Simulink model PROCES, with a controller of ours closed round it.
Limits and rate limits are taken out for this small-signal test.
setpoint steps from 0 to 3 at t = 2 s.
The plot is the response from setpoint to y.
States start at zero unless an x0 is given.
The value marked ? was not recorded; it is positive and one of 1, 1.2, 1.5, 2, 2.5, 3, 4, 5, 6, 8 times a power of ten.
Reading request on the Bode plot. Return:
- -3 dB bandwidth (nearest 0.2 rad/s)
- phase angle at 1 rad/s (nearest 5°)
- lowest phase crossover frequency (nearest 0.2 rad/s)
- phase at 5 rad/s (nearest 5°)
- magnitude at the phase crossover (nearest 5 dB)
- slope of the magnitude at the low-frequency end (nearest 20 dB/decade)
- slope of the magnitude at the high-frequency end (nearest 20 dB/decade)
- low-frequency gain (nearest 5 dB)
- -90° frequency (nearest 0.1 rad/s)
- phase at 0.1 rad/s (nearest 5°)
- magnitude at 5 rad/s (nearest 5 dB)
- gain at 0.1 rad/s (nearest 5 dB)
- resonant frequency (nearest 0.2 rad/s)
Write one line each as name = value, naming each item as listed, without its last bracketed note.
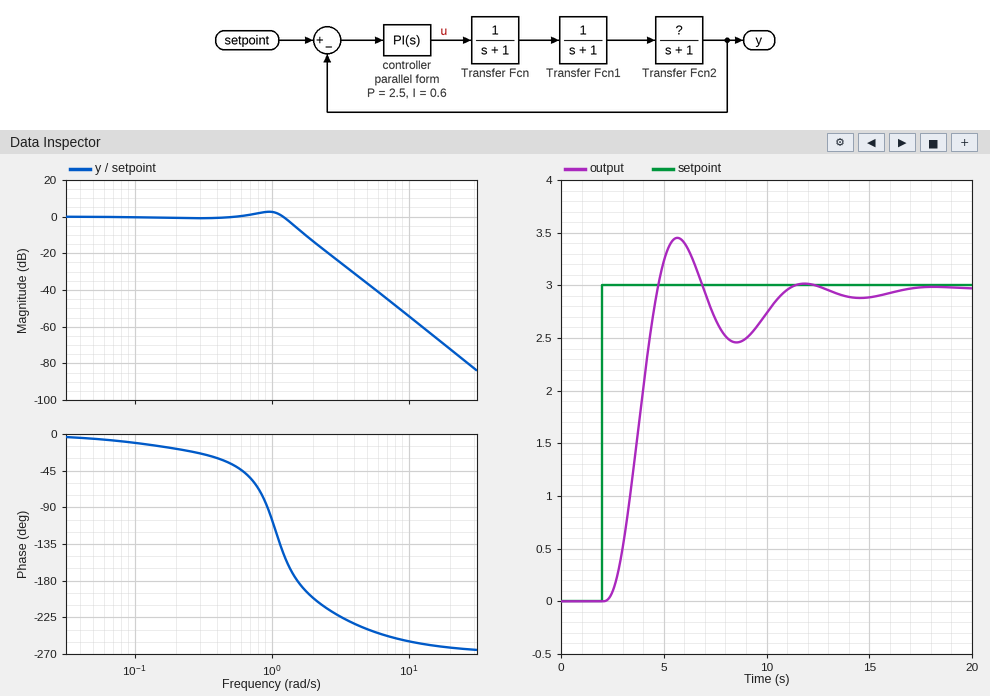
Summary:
-3 dB bandwidth = 1.4 rad/s
phase angle at 1 rad/s = -105°
lowest phase crossover frequency = 1.6 rad/s
phase at 5 rad/s = -240°
magnitude at the phase crossover = -5 dB
slope of the magnitude at the low-frequency end = 0 dB/decade
slope of the magnitude at the high-frequency end = -60 dB/decade
low-frequency gain = 0 dB
-90° frequency = 0.9 rad/s
phase at 0.1 rad/s = -10°
magnitude at 5 rad/s = -35 dB
gain at 0.1 rad/s = 0 dB
resonant frequency = 1.0 rad/s
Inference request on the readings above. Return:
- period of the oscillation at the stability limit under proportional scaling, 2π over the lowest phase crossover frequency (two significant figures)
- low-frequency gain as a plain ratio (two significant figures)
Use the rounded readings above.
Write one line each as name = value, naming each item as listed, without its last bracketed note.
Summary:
period of the oscillation at the stability limit under proportional scaling, 2π over the lowest phase crossover frequency = 3.9 s
low-frequency gain as a plain ratio = 1.0
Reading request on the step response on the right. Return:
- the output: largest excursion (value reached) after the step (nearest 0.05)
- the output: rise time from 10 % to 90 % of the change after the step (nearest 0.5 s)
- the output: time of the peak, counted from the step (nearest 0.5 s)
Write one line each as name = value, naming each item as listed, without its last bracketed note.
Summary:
the output: largest excursion (value reached) after the step = 3.45
the output: rise time from 10 % to 90 % of the change after the step = 1.5 s
the output: time of the peak, counted from the step = 3.5 s
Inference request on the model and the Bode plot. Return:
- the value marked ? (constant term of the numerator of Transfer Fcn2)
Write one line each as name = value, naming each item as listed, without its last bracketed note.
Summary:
the value marked ? = 0.8
